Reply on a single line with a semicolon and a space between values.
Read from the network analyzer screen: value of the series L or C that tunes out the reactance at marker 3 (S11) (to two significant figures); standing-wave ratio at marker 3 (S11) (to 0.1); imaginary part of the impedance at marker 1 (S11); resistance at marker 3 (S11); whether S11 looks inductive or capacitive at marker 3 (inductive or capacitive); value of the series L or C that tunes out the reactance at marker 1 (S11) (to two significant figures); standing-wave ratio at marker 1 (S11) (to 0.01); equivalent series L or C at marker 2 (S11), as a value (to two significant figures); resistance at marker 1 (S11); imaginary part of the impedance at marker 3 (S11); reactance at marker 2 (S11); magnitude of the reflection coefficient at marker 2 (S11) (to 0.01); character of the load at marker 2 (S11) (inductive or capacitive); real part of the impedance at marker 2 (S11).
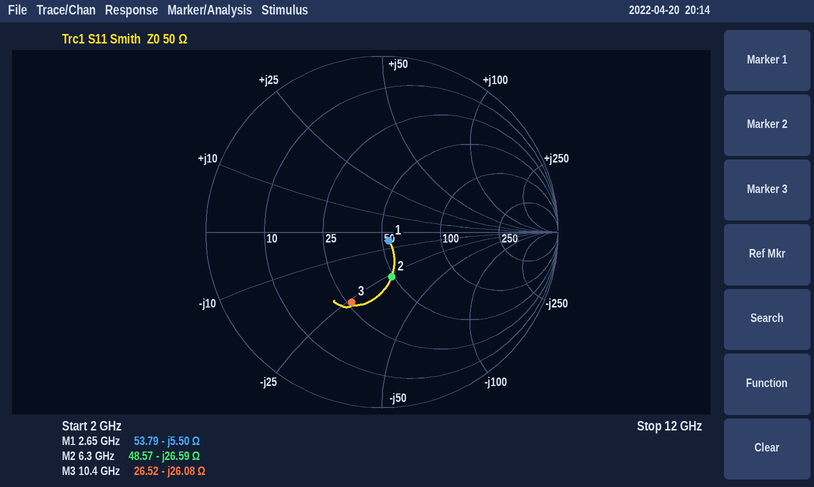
400 pH; 2.5; -5.50 Ω; 26.52 Ω; capacitive; 330 pH; 1.14; 950 fF; 53.79 Ω; -26.08 Ω; -26.59 Ω; 0.26; capacitive; 48.57 Ω
